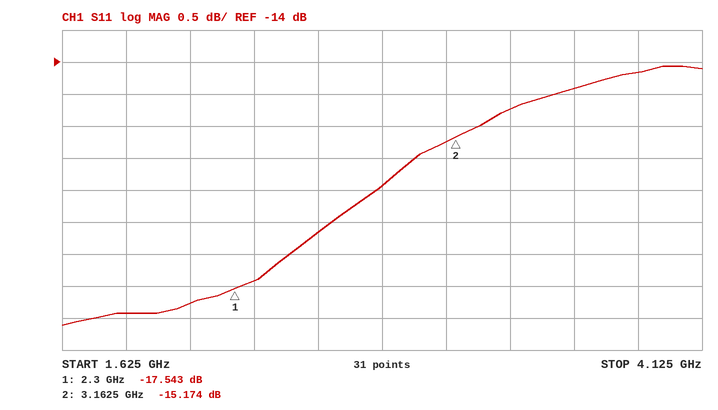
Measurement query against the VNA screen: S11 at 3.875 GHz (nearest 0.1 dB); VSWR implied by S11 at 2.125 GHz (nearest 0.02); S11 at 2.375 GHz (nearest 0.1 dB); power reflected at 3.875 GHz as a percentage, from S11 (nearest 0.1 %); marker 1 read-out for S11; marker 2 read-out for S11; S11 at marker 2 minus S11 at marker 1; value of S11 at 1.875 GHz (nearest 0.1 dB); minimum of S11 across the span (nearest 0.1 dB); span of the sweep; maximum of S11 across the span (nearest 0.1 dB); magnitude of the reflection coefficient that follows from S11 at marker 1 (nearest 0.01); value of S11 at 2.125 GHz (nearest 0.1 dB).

-14.2 dB
1.30
-17.4 dB
3.8 %
-17.543 dB
-15.174 dB
2.369 dB
-17.9 dB
-18.1 dB
2.5 GHz
-14.1 dB
0.13
-17.8 dB
